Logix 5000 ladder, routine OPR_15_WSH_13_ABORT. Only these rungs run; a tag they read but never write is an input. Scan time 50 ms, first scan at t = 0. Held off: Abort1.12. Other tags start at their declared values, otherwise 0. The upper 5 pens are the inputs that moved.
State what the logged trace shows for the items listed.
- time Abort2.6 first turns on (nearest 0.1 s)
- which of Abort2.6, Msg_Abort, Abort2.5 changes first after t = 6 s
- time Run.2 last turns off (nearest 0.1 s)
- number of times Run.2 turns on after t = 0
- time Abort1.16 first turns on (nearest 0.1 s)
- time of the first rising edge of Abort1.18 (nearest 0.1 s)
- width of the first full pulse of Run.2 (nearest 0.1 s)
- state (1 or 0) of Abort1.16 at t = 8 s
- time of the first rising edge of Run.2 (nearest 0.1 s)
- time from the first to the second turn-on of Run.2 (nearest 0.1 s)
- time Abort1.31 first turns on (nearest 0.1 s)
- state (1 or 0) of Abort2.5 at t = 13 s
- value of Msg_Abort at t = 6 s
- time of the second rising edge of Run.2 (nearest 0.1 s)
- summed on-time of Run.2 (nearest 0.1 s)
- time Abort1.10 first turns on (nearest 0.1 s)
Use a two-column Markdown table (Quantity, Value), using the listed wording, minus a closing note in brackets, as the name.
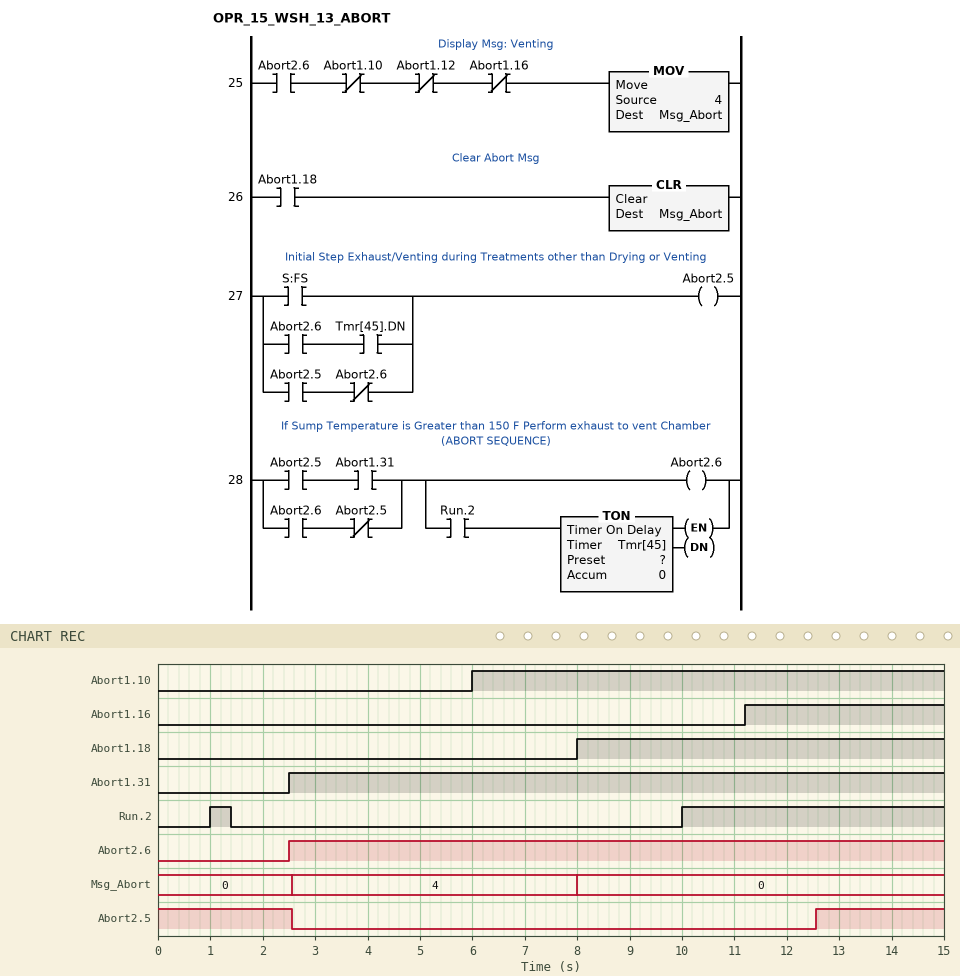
| Quantity | Value |
|---|---|
| time Abort2.6 first turns on | 2.5 s |
| which of Abort2.6, Msg_Abort, Abort2.5 changes first after t = 6 s | Msg_Abort |
| time Run.2 last turns off | 1.4 s |
| number of times Run.2 turns on after t = 0 | 2 |
| time Abort1.16 first turns on | 11.2 s |
| time of the first rising edge of Abort1.18 | 8.0 s |
| width of the first full pulse of Run.2 | 0.4 s |
| state (1 or 0) of Abort1.16 at t = 8 s | 0 |
| time of the first rising edge of Run.2 | 1.0 s |
| time from the first to the second turn-on of Run.2 | 9.0 s |
| time Abort1.31 first turns on | 2.5 s |
| state (1 or 0) of Abort2.5 at t = 13 s | 1 |
| value of Msg_Abort at t = 6 s | 4 |
| time of the second rising edge of Run.2 | 10.0 s |
| summed on-time of Run.2 | 5.4 s |
| time Abort1.10 first turns on | 6.0 s |
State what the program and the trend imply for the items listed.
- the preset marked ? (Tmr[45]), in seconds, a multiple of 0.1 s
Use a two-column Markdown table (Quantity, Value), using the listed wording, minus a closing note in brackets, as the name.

| Quantity | Value |
|---|---|
| the preset marked ? (Tmr[45]), in seconds, a multiple of 0.1 s | 2.5 s |
